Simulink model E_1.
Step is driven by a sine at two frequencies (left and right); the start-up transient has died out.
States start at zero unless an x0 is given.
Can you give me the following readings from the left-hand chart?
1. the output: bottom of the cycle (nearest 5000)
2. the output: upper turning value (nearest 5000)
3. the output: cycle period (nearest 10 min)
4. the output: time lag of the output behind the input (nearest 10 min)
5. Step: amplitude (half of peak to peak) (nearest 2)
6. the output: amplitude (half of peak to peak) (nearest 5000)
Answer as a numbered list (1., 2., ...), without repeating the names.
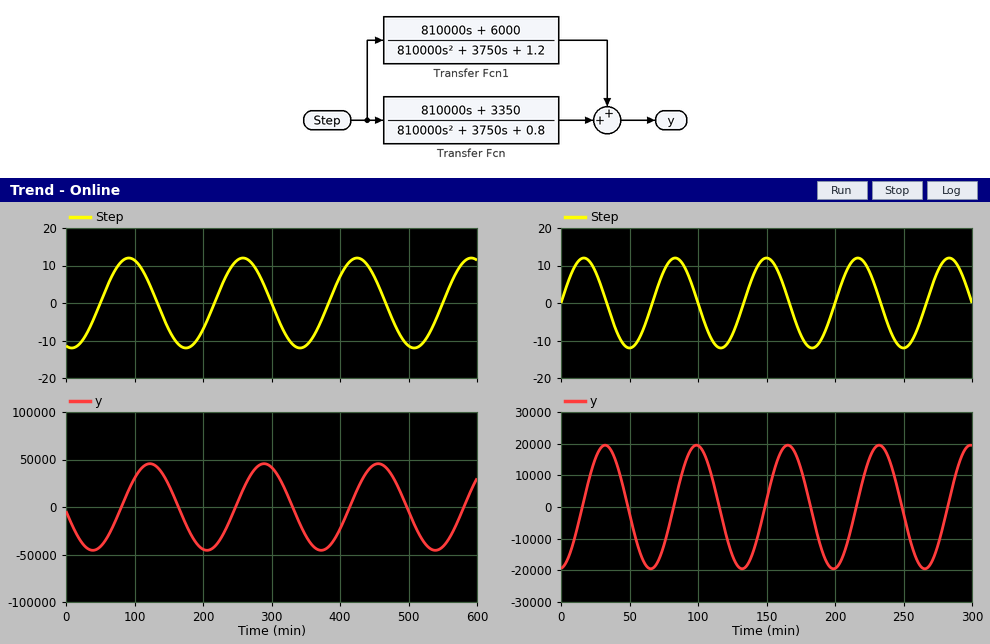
1. -45000
2. 45000
3. 170 min
4. 30 min
5. 12
6. 45000
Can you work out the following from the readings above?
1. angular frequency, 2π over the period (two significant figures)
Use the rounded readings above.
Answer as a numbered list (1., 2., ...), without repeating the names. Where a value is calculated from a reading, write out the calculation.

1. 2π / 170 = 0.037 rad/min
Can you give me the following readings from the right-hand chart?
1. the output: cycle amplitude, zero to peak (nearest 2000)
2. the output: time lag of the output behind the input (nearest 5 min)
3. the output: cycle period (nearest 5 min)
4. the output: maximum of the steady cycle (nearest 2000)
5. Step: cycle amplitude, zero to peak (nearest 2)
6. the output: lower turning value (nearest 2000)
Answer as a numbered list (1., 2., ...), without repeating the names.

1. 20000
2. 15 min
3. 65 min
4. 20000
5. 12
6. -20000
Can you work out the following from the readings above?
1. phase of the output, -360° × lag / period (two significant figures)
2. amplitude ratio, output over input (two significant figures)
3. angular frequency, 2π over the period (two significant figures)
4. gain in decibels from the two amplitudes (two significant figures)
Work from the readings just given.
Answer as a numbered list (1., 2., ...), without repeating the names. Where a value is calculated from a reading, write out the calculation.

1. -360 × 15 / 65 = -83°
2. 20000 / 12 = 1700
3. 2π / 65 = 0.097 rad/min
4. 20 log10(20000 / 12) = 64 dB
